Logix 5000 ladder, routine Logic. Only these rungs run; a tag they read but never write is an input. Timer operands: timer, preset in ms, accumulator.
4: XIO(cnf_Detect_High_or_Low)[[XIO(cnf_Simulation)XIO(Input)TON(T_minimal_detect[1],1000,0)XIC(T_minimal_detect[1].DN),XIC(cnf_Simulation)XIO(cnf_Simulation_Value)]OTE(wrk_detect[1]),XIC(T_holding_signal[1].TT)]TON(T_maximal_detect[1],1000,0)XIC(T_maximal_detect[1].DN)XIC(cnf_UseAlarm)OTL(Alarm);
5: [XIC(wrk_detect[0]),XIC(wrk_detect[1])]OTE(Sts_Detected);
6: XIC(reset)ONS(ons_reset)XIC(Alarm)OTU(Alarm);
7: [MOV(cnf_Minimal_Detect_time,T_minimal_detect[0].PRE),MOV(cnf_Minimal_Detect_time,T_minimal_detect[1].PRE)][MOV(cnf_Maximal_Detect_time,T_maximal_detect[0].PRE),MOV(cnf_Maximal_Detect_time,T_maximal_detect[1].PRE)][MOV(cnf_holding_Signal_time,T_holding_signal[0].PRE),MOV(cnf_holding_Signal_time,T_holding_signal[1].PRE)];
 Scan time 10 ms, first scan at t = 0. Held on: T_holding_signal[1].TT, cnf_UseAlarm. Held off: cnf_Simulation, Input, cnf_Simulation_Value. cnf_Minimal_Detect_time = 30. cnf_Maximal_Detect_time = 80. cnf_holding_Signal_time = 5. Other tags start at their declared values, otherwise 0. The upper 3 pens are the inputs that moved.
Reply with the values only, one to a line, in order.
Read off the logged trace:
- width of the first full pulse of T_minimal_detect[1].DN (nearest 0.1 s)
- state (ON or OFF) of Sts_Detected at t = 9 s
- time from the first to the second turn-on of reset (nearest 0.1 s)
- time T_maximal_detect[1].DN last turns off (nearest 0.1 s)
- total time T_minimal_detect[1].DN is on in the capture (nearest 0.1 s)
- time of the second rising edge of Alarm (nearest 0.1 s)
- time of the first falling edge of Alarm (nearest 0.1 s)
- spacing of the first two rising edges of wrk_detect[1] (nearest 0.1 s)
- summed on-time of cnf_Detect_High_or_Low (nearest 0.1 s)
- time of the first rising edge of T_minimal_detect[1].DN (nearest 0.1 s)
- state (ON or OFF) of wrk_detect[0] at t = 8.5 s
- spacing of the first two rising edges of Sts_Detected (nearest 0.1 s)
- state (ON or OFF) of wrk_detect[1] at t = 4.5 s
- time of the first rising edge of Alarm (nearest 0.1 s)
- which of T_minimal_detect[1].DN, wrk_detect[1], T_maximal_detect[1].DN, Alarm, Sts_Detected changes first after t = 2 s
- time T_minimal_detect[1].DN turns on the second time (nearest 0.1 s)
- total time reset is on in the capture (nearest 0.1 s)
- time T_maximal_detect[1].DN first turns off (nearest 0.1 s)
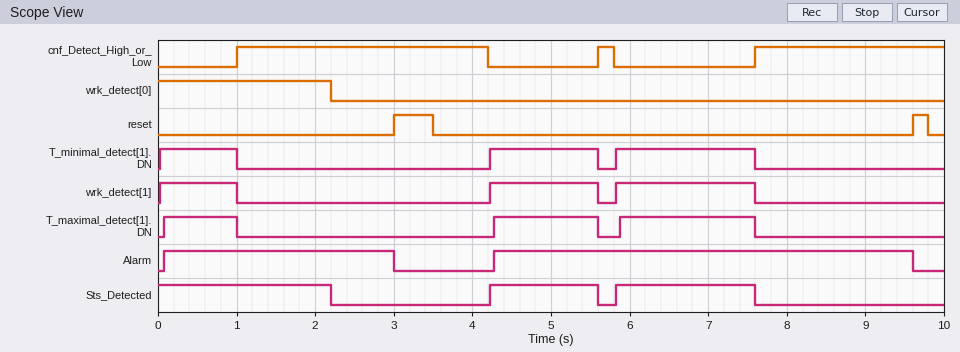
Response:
1.0 s
OFF
6.6 s
7.6 s
4.1 s
4.3 s
3.0 s
4.2 s
5.8 s
0.0 s
OFF
1.6 s
ON
0.1 s
Sts_Detected
4.2 s
0.7 s
1.0 s
